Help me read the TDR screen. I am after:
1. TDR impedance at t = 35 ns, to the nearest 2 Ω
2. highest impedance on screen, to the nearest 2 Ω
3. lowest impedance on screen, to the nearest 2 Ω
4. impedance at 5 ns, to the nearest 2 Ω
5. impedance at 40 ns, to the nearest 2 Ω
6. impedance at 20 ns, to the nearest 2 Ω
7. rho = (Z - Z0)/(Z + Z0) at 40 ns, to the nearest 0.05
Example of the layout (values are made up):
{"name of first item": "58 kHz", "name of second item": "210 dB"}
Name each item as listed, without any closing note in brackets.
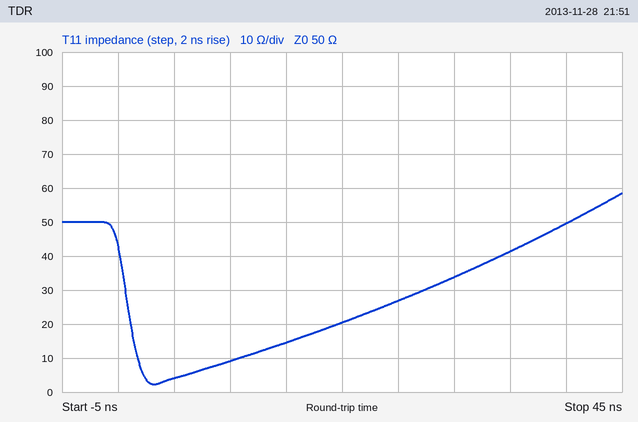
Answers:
{"TDR impedance at t = 35 ns, to the nearest 2 Ω": "42 Ω", "highest impedance on screen, to the nearest 2 Ω": "58 Ω", "lowest impedance on screen, to the nearest 2 Ω": "2 Ω", "impedance at 5 ns, to the nearest 2 Ω": "4 Ω", "impedance at 40 ns, to the nearest 2 Ω": "50 Ω", "impedance at 20 ns, to the nearest 2 Ω": "20 Ω", "rho = (Z - Z0)/(Z + Z0) at 40 ns, to the nearest 0.05": "0.00"}
